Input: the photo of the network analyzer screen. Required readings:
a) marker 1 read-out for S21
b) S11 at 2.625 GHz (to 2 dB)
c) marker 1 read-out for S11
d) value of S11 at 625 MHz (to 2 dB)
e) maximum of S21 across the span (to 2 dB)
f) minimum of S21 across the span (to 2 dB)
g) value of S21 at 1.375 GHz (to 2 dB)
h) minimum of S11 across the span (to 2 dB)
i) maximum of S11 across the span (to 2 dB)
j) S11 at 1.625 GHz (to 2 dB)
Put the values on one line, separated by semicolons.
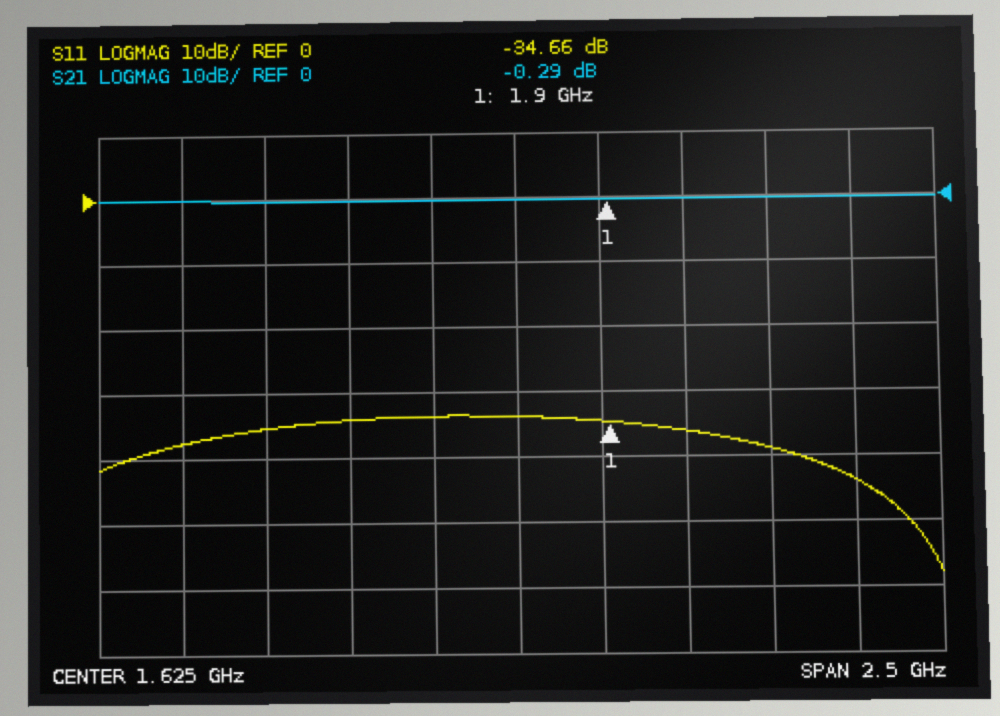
-0.29 dB; -44 dB; -34.66 dB; -38 dB; 0 dB; 0 dB; 0 dB; -58 dB; -34 dB; -34 dB
